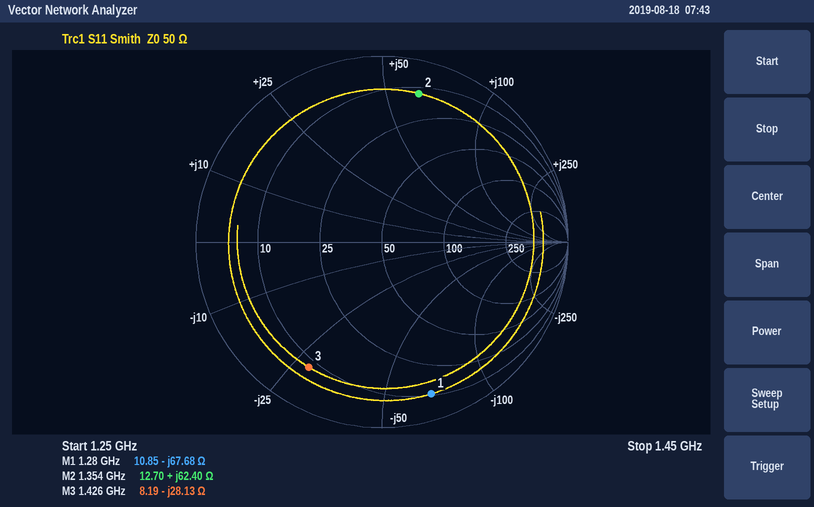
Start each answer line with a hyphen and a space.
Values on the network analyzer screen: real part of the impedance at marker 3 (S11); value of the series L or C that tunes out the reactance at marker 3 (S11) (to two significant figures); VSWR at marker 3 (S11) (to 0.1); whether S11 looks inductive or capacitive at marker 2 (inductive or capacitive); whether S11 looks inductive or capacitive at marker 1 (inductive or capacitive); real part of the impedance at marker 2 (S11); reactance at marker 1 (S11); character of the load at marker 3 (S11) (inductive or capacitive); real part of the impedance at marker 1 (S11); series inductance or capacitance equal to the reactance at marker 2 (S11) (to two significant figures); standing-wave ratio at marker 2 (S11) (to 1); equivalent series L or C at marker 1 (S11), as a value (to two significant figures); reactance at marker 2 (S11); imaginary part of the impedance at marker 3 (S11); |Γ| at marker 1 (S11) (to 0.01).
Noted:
- 8.19 Ω
- 3.1 nH
- 8.1
- inductive
- capacitive
- 12.70 Ω
- -67.68 Ω
- capacitive
- 10.85 Ω
- 7.3 nH
- 10
- 1.8 pF
- +62.40 Ω
- -28.13 Ω
- 0.86
